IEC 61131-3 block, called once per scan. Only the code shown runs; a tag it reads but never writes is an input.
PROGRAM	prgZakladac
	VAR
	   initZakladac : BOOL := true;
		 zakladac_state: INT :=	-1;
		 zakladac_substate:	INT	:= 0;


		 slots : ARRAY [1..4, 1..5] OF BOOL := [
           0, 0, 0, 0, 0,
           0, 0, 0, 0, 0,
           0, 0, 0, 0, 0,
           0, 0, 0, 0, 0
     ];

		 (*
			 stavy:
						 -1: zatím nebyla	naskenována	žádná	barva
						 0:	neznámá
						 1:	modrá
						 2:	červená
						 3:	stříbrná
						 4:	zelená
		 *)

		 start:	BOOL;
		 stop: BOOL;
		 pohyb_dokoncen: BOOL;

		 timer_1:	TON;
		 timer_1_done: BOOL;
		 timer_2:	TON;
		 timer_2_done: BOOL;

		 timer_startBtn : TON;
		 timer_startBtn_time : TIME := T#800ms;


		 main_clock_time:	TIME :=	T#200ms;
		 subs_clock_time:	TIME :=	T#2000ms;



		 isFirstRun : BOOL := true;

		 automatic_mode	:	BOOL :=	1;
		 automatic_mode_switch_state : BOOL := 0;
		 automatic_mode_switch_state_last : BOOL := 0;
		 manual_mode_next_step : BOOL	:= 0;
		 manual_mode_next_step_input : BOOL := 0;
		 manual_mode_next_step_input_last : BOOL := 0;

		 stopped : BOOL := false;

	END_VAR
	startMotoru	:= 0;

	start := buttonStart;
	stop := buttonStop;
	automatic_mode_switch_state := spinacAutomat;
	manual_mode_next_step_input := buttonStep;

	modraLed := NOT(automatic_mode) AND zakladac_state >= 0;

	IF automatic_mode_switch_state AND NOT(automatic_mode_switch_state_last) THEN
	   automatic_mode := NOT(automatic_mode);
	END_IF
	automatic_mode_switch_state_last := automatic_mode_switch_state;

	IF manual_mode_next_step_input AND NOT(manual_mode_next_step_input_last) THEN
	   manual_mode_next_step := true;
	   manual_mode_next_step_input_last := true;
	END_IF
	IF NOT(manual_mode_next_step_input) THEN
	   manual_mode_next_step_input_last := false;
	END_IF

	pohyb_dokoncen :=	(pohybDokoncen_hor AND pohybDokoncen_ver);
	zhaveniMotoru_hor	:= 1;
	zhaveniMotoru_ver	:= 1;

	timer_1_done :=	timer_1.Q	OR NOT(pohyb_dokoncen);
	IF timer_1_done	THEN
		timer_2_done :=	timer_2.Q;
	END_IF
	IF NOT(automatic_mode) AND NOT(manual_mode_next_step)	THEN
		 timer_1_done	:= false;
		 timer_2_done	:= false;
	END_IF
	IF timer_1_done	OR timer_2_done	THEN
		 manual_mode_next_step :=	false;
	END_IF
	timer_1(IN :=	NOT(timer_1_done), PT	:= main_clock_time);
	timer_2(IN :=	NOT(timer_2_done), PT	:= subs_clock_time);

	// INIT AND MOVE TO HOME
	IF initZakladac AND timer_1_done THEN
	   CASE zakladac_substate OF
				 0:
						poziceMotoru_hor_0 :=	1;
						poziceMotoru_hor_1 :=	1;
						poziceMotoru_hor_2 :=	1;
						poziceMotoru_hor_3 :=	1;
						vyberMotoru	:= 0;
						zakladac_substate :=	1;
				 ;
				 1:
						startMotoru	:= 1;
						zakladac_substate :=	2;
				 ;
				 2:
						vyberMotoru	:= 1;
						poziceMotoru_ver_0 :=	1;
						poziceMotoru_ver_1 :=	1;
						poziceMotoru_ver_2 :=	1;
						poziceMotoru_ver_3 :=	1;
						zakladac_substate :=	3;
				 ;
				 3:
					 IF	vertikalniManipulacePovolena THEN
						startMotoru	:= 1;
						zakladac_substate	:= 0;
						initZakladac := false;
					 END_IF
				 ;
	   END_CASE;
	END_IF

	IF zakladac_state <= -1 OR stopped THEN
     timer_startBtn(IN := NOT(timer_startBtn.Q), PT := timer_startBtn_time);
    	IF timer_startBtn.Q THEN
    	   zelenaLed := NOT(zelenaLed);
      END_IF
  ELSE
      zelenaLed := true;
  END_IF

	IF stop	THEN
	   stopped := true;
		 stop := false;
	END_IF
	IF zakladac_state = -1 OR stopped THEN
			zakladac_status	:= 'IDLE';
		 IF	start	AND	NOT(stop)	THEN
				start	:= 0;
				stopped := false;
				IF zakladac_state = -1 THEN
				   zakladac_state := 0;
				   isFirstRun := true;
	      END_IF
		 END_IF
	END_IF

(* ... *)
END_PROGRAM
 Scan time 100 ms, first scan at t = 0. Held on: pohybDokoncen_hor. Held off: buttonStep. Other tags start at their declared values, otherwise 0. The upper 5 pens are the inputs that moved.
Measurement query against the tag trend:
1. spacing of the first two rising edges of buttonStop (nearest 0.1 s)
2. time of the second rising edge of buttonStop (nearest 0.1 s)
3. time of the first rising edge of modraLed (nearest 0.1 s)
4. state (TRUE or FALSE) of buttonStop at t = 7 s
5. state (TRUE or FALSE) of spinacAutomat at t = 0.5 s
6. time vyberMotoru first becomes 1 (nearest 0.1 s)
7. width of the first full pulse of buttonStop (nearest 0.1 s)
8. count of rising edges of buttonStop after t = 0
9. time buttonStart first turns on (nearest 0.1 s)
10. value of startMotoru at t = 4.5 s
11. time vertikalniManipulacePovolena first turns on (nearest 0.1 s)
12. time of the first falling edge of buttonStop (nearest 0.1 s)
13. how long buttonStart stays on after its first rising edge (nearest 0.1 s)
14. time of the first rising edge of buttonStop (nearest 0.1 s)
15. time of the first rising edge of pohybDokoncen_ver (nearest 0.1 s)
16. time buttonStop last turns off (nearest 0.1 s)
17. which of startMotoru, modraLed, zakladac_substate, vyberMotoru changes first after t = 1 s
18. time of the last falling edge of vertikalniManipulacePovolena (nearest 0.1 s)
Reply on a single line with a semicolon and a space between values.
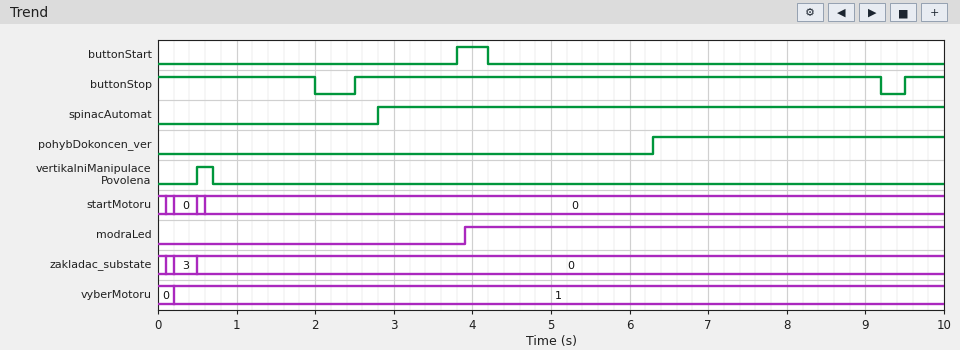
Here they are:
7.0 s; 9.5 s; 3.9 s; TRUE; FALSE; 0.2 s; 6.7 s; 2; 3.8 s; 0; 0.5 s; 2.0 s; 0.4 s; 2.5 s; 6.3 s; 9.2 s; modraLed; 0.7 s
